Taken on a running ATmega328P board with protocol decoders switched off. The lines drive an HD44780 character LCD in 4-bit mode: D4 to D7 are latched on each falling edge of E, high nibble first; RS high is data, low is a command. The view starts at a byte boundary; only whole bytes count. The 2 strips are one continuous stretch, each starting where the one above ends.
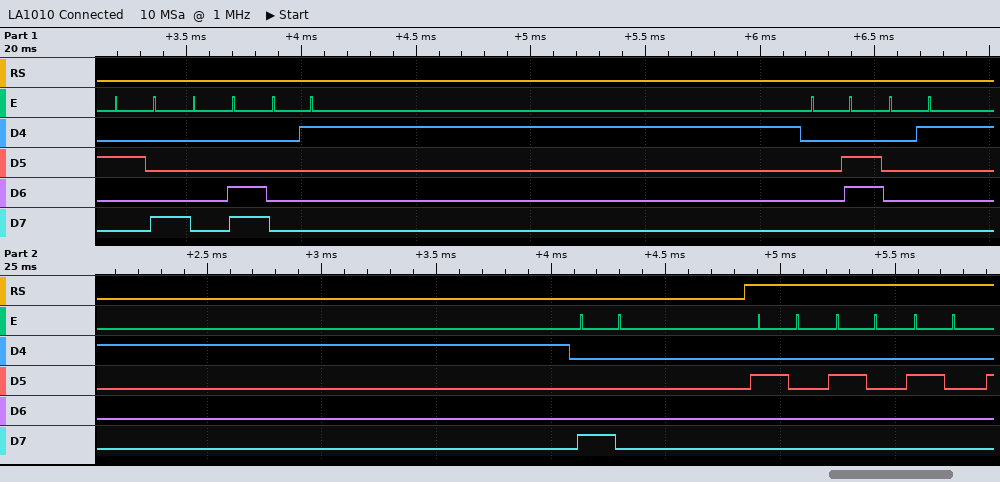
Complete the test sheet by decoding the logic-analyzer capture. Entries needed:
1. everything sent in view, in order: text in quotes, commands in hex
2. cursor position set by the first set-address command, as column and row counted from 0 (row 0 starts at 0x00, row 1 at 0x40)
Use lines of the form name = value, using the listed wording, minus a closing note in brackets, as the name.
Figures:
everything sent in view, in order: text in quotes, commands in hex = 0x28 0x0C 0x01 0x06 0x01 0x80 "   "
cursor position set by the first set-address command, as column and row counted from 0 = column 0, row 0
